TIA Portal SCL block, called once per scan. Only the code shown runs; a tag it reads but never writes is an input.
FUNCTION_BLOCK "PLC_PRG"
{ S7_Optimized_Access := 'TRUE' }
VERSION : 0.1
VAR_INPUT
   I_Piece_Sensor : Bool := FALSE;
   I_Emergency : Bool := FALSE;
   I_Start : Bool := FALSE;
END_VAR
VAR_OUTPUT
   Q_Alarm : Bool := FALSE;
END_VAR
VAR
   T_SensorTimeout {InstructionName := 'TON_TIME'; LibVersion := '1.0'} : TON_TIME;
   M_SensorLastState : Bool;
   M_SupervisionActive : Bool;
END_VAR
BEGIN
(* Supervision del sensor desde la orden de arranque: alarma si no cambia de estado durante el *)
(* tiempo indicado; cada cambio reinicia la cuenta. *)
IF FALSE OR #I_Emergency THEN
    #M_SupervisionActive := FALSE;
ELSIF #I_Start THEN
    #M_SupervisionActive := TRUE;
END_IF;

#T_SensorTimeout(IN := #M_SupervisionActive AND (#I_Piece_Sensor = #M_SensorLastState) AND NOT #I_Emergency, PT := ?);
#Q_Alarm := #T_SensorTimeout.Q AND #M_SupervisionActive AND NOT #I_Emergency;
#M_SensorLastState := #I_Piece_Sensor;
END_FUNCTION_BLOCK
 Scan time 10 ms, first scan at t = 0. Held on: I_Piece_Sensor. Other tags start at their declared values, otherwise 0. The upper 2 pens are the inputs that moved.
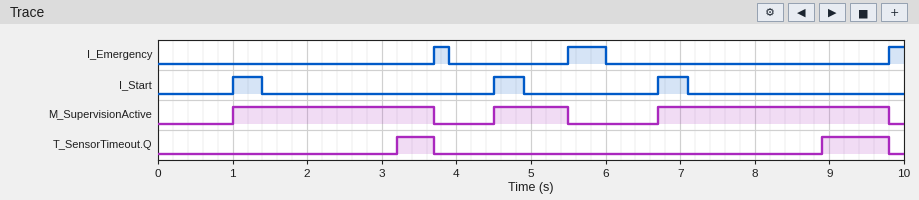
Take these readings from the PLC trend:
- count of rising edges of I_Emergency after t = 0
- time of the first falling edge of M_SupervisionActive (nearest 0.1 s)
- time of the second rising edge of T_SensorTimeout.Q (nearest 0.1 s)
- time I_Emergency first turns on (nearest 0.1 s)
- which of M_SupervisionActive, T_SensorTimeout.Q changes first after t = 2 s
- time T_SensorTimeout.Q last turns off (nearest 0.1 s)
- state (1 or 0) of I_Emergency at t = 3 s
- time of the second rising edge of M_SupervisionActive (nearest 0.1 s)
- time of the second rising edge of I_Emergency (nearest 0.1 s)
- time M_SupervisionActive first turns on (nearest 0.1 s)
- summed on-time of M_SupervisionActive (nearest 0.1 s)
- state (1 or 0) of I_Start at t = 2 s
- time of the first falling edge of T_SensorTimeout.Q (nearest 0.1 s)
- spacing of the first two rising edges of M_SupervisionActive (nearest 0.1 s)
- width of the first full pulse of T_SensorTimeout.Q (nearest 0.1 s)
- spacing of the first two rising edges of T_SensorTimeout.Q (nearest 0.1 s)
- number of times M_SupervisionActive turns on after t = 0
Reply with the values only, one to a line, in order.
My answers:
3
3.7 s
8.9 s
3.7 s
T_SensorTimeout.Q
9.8 s
0
4.5 s
5.5 s
1.0 s
6.8 s
0
3.7 s
3.5 s
0.5 s
5.7 s
3
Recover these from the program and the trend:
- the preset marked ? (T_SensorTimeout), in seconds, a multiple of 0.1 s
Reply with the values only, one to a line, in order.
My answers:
2.2 s
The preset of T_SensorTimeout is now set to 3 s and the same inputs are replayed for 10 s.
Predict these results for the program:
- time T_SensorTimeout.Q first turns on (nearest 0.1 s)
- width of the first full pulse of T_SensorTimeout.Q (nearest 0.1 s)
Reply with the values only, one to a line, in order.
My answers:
9.7 s
0.1 s
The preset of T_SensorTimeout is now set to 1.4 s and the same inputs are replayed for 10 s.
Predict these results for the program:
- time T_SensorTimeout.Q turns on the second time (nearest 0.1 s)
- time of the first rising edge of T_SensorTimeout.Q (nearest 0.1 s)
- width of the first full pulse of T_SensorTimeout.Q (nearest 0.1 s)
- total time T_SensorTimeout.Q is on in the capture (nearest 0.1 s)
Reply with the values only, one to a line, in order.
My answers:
8.1 s
2.4 s
1.3 s
3.0 s
